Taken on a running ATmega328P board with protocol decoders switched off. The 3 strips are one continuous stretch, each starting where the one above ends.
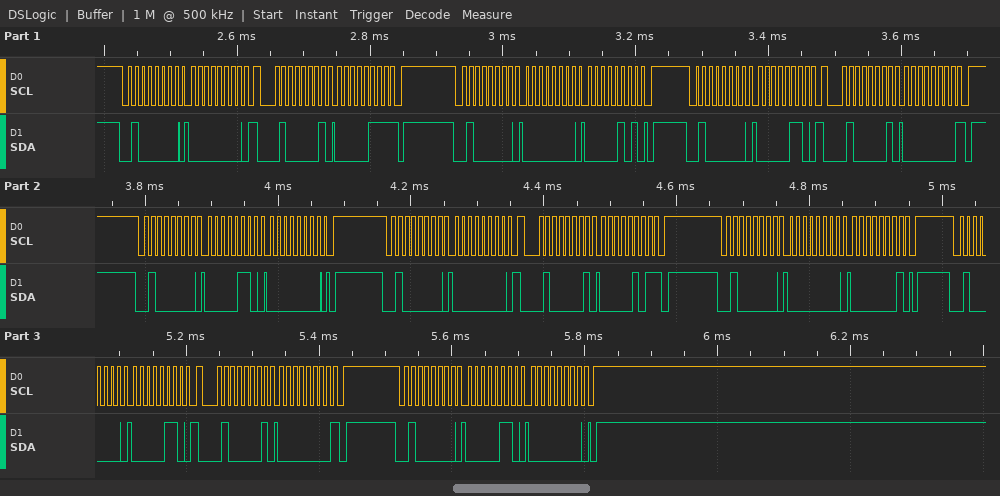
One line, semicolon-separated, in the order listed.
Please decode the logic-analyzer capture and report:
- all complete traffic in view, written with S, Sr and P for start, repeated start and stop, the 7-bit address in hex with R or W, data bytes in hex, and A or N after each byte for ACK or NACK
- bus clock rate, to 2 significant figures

S 20W A 00 A Sr 20R A 07 N P S 20W A 00 A 05 A P S 20W A 06 A Sr 20R A 00 N P S 20W A 06 A 00 A P S 20W A 00 A Sr 20R A 05 N P S 20W A 00 A 01 A P S 20W A 06 A Sr 20R A 00 N P S 20W A 06 A 00 A P; 100 kHz
